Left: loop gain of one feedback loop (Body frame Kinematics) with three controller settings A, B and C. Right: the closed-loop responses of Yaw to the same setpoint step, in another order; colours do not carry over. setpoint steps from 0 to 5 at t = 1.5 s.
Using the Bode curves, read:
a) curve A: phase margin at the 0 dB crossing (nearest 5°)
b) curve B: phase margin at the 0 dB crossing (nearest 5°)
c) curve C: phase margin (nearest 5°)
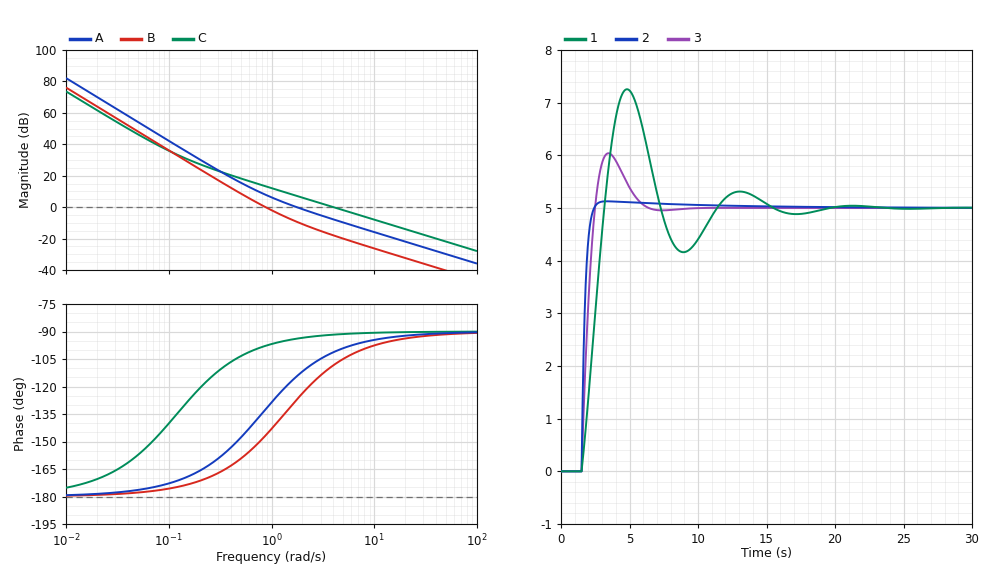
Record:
65°
35°
90°
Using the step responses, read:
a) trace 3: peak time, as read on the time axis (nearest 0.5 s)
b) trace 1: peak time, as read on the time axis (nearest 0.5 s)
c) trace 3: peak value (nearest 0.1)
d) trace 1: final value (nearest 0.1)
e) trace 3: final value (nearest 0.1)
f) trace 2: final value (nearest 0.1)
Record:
3.5 s
5.0 s
6.0
5.0
5.0
5.0
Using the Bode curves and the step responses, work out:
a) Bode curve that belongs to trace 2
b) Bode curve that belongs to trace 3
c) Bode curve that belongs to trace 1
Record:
C
A
B
